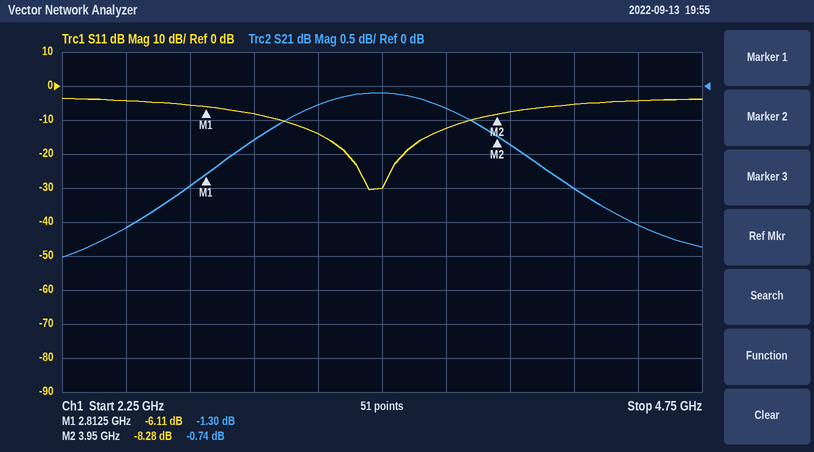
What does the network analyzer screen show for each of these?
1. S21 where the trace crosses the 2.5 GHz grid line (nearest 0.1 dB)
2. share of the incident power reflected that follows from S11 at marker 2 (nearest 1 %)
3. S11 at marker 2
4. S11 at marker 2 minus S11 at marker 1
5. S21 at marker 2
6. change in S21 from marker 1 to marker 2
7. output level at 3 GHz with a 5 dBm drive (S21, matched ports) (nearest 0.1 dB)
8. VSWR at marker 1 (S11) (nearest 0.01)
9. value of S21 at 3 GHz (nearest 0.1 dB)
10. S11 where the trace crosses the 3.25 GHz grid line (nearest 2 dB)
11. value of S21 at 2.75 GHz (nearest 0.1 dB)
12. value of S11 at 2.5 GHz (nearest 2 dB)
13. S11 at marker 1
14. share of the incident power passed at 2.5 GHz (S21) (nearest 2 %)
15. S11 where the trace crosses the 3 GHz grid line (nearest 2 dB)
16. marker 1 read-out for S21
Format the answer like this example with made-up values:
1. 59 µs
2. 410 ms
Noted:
1. -2.1 dB
2. 15 %
3. -8.28 dB
4. -2.17 dB
5. -0.74 dB
6. 0.56 dB
7. 4.2 dBm
8. 2.96
9. -0.8 dB
10. -14 dB
11. -1.5 dB
12. -4 dB
13. -6.11 dB
14. 62 %
15. -8 dB
16. -1.30 dB
